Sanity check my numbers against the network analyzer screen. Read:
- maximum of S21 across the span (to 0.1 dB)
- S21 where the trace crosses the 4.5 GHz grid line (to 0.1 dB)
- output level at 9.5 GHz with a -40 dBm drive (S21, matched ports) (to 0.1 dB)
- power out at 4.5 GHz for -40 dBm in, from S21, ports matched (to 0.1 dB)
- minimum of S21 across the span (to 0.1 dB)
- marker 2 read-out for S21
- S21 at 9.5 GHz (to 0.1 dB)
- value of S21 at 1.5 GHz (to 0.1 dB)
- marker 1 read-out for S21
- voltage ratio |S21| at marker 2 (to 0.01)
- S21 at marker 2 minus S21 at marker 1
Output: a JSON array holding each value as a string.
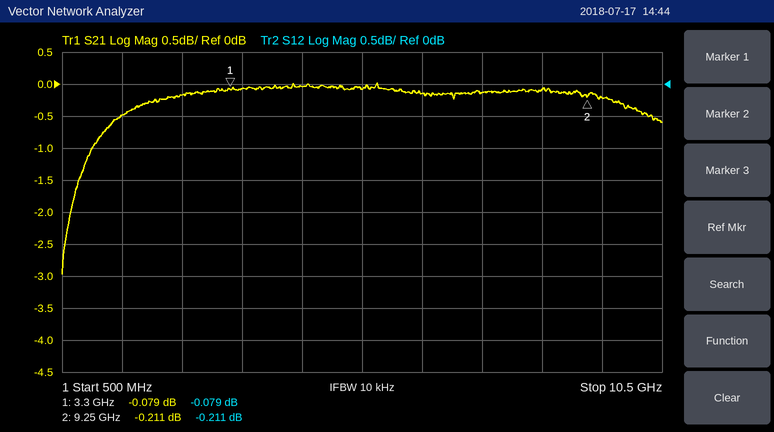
["0.0 dB", "0.0 dB", "-40.2 dBm", "-40.0 dBm", "-3.0 dB", "-0.211 dB", "-0.2 dB", "-0.5 dB", "-0.079 dB", "0.98", "-0.132 dB"]
